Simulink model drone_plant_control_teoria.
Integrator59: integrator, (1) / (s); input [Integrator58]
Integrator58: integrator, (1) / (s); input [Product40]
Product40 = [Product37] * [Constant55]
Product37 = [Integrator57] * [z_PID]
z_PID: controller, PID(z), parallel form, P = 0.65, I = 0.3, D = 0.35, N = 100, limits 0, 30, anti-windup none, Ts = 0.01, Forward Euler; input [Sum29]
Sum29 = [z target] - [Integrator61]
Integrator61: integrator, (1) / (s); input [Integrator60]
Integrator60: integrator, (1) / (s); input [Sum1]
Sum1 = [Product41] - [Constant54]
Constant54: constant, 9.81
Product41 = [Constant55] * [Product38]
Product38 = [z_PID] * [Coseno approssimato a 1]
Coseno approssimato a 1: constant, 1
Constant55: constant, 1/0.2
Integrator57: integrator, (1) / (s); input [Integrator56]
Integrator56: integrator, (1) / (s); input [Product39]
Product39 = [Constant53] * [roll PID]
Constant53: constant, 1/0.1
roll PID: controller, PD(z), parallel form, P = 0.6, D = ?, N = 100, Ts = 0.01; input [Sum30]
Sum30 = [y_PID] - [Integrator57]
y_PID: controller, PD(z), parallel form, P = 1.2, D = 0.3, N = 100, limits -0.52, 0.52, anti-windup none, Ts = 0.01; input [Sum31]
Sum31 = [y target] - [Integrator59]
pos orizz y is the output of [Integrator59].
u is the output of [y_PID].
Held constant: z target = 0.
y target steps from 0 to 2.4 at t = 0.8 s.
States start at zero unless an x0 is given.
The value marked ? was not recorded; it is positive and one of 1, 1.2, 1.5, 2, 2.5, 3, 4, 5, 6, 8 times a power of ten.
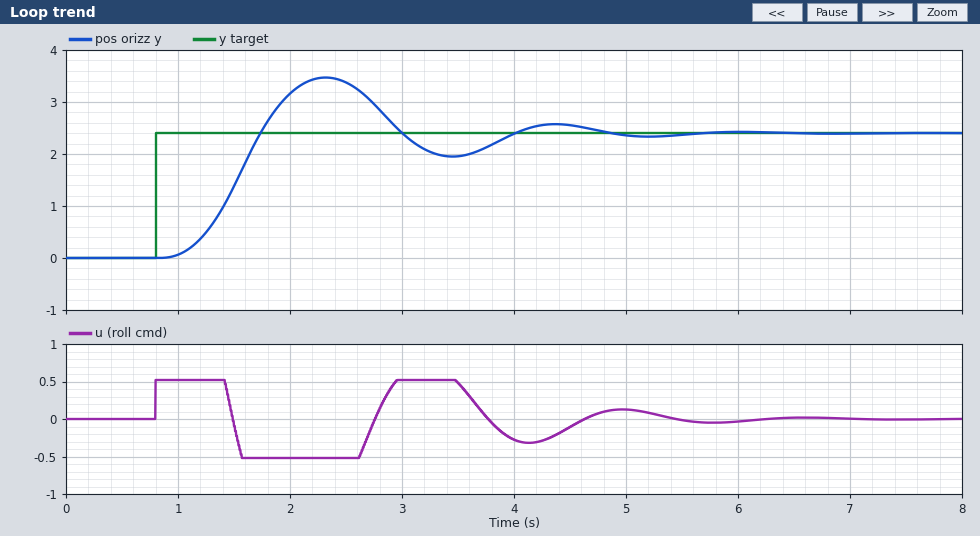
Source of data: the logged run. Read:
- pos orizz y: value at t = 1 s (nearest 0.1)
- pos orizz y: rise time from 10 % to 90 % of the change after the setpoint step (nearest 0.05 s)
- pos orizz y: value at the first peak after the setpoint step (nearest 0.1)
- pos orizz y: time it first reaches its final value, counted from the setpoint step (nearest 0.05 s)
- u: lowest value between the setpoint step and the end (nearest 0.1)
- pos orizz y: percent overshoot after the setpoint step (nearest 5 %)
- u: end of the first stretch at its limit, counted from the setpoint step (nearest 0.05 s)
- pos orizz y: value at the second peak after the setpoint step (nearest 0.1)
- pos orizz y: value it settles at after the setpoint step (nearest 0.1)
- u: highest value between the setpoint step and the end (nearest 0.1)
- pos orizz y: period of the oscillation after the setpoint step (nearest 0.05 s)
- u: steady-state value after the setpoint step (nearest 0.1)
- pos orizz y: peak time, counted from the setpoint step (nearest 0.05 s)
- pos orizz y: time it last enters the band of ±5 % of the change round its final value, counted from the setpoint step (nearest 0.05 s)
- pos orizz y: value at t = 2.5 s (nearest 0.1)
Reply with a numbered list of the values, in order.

1. 0.1
2. 0.55 s
3. 3.5
4. 0.95 s
5. -0.5
6. 45 %
7. 0.60 s
8. 2.6
9. 2.4
10. 0.5
11. 2.05 s
12. 0.0
13. 1.50 s
14. 3.80 s
15. 3.4
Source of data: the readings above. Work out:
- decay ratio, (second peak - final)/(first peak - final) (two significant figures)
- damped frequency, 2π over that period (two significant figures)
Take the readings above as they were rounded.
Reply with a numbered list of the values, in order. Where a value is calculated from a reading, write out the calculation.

1. (2.6 - 2.4) / (3.5 - 2.4) = 0.18
2. 2π / 2.05 = 3.1 rad/s
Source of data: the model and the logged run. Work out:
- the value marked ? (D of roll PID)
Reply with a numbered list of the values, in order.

1. 1.2
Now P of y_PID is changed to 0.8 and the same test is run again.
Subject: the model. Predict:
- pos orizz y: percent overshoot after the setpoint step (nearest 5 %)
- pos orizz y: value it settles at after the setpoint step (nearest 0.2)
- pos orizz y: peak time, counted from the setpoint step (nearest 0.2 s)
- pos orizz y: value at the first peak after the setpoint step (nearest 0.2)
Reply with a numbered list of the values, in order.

1. 15 %
2. 2.4
3. 1.4 s
4. 2.8
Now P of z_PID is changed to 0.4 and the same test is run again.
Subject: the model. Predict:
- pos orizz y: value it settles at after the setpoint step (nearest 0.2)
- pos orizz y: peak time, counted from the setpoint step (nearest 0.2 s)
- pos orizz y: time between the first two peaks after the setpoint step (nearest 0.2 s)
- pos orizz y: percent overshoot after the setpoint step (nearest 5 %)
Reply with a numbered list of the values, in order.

1. 2.4
2. 1.4 s
3. 1.8 s
4. 40 %
